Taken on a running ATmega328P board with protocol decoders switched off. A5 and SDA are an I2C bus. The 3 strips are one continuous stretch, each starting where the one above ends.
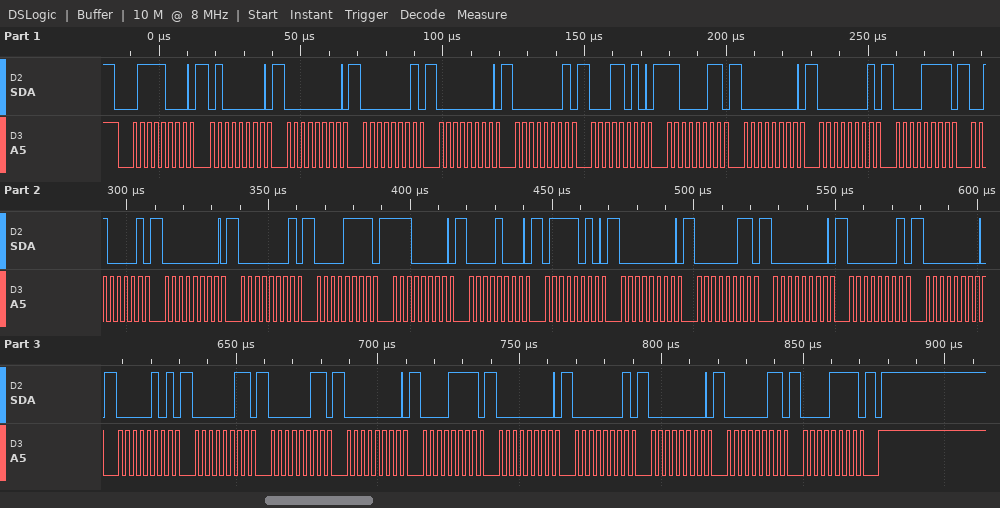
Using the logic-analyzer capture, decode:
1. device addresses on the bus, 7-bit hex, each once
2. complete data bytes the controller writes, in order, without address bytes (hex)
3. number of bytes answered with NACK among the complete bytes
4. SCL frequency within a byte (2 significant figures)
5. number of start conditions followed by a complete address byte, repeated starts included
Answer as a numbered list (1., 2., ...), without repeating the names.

1. 0x3C
2. 40 00 01 00 01 1A C3 00 01 0F 21 00 01 0F E0 08 7A 00 03 00 01 00 05 03 03 00 0F 00 01 00 03 0F
3. 0
4. 400 kHz
5. 1
